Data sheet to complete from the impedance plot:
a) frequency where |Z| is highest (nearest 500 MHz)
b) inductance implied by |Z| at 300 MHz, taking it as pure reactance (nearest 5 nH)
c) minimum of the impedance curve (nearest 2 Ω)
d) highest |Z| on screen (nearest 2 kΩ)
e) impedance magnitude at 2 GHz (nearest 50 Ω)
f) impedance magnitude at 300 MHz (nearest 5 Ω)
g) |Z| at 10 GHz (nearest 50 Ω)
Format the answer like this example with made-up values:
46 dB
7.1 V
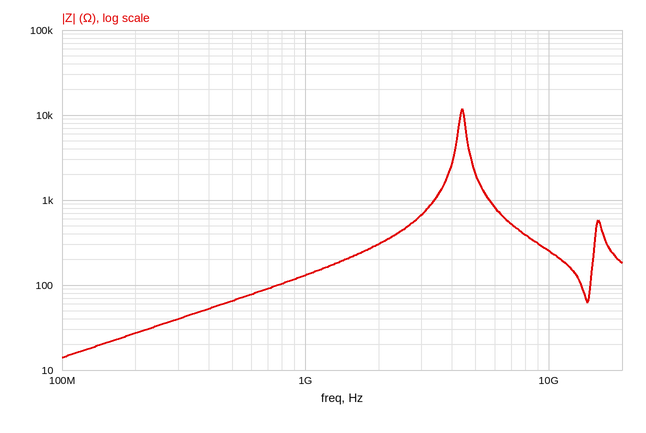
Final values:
4.5 GHz
20 nH
14 Ω
12 kΩ
300 Ω
40 Ω
250 Ω
